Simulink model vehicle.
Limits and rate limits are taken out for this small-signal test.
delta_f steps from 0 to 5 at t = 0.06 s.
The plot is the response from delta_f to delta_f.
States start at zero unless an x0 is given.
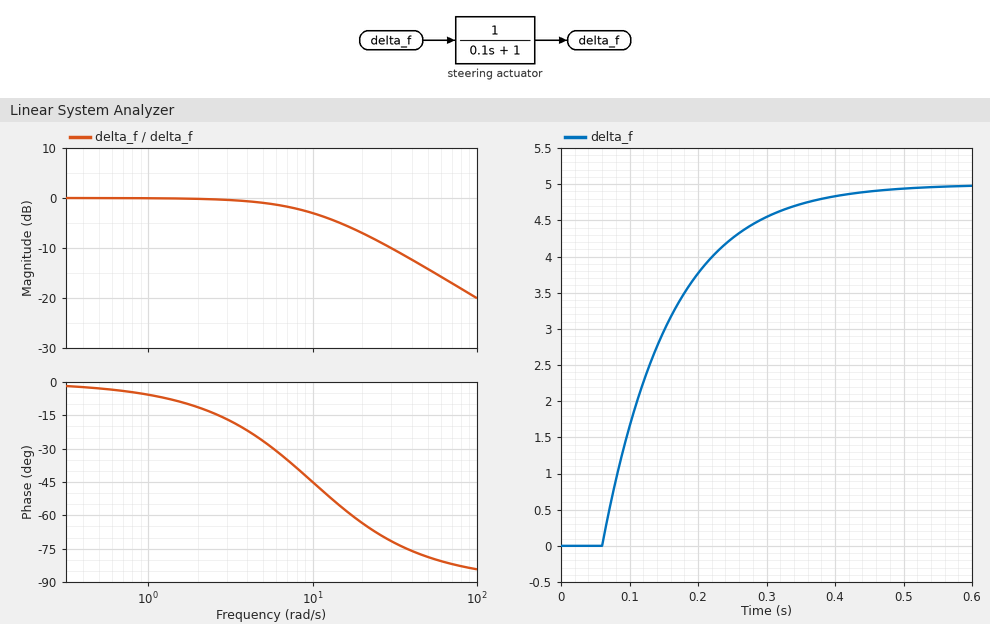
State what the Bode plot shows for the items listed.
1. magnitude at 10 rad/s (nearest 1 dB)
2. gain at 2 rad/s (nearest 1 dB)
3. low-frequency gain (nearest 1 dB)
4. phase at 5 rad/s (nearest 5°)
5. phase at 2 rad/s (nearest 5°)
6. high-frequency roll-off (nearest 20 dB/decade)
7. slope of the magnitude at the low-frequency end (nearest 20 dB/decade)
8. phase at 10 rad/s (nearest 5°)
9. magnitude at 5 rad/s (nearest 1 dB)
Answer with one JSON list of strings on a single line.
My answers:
["-3 dB", "0 dB", "0 dB", "-25°", "-10°", "-20 dB/decade", "0 dB/decade", "-45°", "-1 dB"]
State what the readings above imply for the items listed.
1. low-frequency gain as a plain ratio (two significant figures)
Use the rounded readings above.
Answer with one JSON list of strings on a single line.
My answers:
["1.0"]
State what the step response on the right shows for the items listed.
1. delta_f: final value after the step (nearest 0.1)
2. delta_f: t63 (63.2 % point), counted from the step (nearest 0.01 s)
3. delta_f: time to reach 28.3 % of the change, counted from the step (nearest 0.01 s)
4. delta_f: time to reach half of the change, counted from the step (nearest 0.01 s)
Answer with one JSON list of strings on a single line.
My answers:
["5.0", "0.10 s", "0.03 s", "0.07 s"]
